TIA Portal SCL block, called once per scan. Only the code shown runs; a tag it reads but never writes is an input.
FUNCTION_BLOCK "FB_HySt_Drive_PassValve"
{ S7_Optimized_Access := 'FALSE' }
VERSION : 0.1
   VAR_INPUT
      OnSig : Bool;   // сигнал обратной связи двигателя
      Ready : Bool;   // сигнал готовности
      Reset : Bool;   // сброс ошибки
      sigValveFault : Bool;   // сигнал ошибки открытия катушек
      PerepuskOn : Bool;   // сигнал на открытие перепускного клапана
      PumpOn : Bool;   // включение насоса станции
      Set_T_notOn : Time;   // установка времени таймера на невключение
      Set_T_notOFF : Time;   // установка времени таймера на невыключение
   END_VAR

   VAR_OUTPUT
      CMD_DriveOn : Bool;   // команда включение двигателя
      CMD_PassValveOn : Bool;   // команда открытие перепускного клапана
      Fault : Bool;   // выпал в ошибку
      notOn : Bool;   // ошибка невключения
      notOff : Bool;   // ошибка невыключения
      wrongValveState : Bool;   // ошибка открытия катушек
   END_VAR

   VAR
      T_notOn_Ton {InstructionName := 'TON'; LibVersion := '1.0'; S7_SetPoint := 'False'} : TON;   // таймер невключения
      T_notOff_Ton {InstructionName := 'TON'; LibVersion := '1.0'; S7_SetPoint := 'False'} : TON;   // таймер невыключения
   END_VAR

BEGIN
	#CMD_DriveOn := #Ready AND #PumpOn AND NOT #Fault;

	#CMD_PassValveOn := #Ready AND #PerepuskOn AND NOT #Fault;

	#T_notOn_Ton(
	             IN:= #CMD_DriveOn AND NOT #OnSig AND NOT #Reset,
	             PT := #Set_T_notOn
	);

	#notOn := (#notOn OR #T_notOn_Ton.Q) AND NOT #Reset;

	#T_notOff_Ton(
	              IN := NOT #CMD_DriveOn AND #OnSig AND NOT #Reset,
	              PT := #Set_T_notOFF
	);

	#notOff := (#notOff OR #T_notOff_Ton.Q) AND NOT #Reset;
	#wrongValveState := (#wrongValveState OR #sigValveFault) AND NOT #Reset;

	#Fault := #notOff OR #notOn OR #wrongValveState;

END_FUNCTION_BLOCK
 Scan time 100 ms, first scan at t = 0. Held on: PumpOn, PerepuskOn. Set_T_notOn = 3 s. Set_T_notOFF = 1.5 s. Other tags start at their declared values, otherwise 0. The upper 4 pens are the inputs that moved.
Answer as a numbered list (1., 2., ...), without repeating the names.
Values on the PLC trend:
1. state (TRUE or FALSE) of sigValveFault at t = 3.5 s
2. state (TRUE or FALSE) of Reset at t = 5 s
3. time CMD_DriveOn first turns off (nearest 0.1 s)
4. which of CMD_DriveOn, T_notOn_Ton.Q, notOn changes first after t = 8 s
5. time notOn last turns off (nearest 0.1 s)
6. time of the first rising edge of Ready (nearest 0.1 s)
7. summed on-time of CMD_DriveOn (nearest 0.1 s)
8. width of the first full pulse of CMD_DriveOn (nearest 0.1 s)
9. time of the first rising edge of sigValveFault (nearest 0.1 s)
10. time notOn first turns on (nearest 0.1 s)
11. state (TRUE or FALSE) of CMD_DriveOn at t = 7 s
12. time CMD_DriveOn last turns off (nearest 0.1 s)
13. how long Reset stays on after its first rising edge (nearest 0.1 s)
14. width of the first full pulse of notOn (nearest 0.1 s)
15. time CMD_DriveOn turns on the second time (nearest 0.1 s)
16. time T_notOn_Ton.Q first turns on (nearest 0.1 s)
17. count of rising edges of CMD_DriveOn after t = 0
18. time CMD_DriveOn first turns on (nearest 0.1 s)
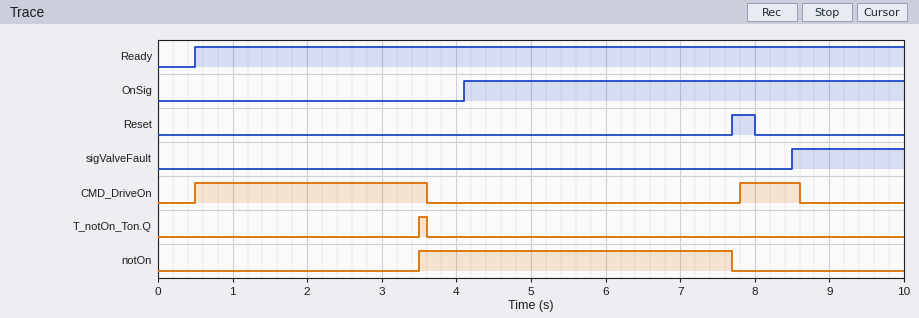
1. FALSE
2. FALSE
3. 3.6 s
4. CMD_DriveOn
5. 7.7 s
6. 0.5 s
7. 3.9 s
8. 3.1 s
9. 8.5 s
10. 3.5 s
11. FALSE
12. 8.6 s
13. 0.3 s
14. 4.2 s
15. 7.8 s
16. 3.5 s
17. 2
18. 0.5 s
